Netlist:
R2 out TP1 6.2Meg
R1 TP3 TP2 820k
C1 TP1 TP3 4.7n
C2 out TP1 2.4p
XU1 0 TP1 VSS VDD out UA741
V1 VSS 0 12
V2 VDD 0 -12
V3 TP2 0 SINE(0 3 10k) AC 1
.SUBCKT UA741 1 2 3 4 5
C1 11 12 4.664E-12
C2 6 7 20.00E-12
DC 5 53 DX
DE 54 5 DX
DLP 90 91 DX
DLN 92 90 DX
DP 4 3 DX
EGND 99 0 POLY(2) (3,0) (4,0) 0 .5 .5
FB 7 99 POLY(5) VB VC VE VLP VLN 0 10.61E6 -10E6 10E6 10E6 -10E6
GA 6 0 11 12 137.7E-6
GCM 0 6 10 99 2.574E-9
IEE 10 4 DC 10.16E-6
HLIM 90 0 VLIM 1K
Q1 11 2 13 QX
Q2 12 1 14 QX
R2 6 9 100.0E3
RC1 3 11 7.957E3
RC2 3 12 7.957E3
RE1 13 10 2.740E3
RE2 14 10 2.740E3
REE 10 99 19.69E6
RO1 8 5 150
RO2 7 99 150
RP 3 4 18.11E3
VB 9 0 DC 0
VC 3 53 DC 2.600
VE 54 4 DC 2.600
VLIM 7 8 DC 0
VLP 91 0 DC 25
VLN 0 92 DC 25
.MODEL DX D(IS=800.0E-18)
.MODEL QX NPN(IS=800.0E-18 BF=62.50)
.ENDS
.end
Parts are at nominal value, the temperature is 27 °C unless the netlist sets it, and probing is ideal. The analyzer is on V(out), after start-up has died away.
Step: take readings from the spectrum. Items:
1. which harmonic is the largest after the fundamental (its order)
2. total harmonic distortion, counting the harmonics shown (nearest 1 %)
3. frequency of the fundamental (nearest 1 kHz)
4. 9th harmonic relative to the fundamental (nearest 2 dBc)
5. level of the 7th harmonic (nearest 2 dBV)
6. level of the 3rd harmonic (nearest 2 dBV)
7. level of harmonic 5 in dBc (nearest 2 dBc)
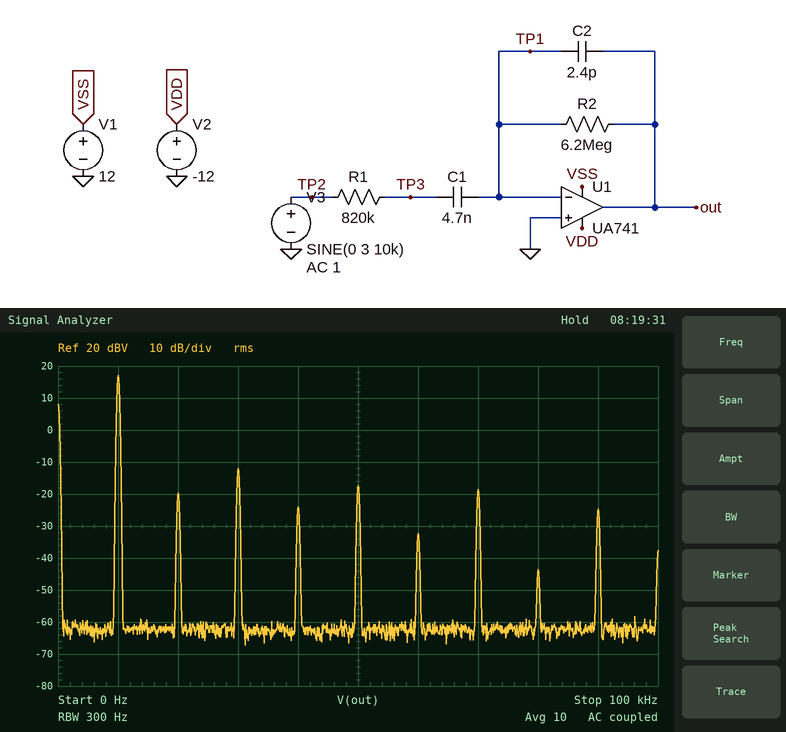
3
5 %
10 kHz
-42 dBc
-18 dBV
-12 dBV
-34 dBc
